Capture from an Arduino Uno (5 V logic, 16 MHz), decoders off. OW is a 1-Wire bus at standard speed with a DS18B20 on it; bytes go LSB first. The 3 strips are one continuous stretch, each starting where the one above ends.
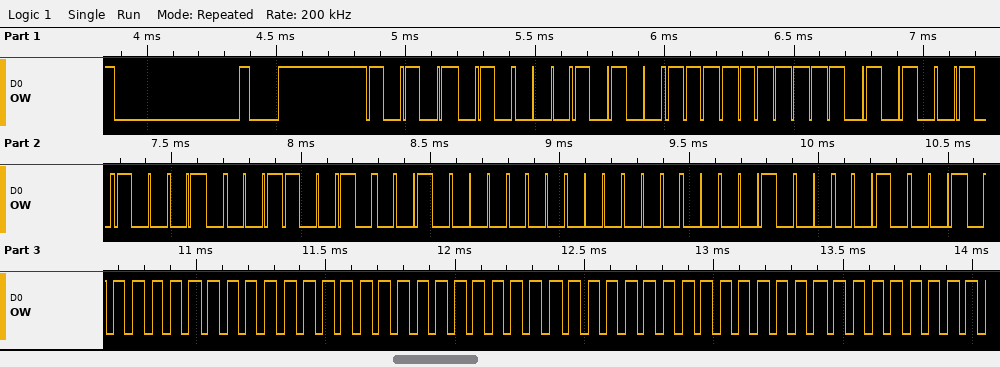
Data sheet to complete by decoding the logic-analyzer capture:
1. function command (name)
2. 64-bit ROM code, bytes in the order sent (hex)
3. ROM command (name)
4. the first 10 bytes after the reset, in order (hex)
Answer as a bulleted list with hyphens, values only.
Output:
- Convert T
- 28 FF 2B 45 4C 04 00 10
- Match ROM
- 55 28 FF 2B 45 4C 04 00 10 44
